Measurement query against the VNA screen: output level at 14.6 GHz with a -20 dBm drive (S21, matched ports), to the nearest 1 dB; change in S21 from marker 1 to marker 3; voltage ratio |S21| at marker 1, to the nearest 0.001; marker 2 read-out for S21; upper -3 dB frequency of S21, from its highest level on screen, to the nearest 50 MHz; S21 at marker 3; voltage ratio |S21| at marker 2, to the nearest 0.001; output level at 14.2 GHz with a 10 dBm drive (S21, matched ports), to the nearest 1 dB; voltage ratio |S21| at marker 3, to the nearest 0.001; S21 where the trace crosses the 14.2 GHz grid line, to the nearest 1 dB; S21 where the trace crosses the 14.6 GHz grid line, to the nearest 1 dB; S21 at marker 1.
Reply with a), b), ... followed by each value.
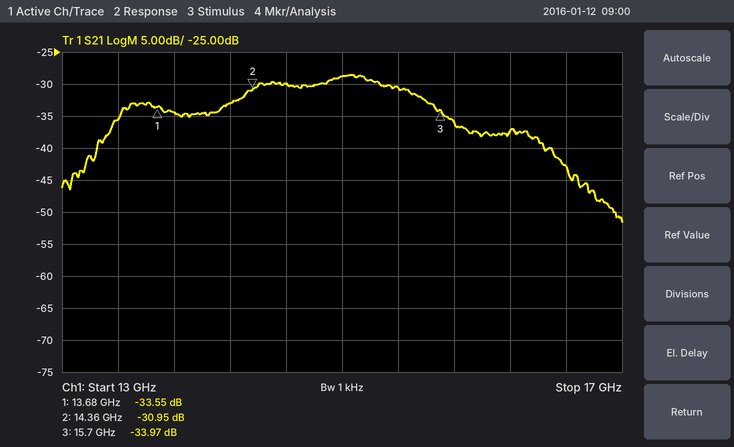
a) -50 dBm
b) -0.42 dB
c) 0.021
d) -30.95 dB
e) 15.50 GHz
f) -33.97 dB
g) 0.028
h) -23 dBm
i) 0.020
j) -33 dB
k) -30 dB
l) -33.55 dB
